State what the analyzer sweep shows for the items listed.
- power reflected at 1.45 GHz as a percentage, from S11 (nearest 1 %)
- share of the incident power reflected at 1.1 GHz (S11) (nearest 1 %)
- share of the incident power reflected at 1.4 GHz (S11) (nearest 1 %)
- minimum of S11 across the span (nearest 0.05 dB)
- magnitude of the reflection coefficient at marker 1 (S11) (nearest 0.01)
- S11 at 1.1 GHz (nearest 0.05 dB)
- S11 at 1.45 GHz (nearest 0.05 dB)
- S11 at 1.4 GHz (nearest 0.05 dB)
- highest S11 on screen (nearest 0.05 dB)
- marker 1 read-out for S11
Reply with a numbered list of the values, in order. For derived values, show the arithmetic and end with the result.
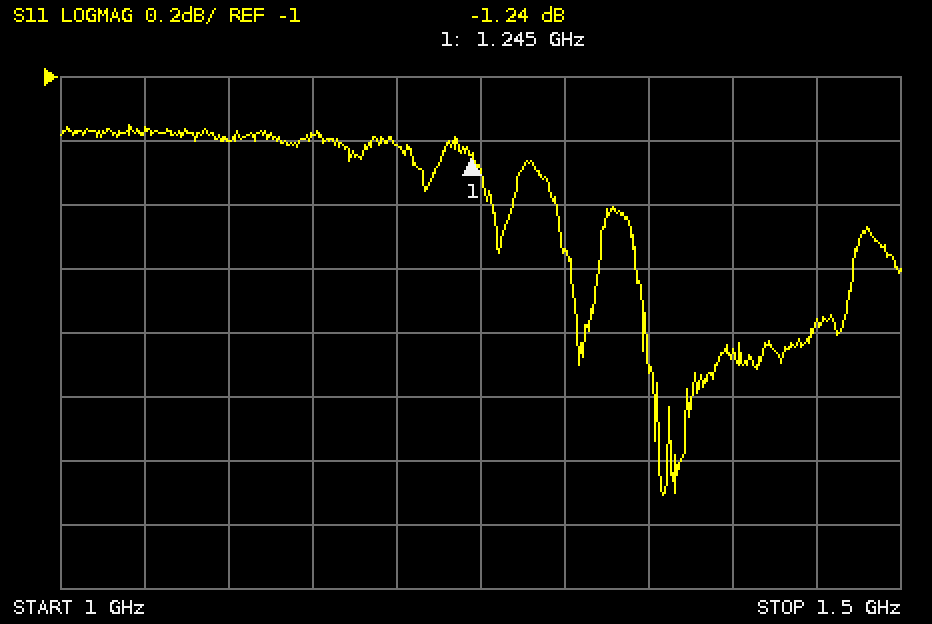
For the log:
1. 10^(-1.75/10) ≈ 67 %
2. 10^(-1.2/10) ≈ 76 %
3. 10^(-1.85/10) ≈ 65 %
4. -2.30 dB
5. 10^(-1.24/20) ≈ 0.87
6. -1.20 dB
7. -1.75 dB
8. -1.85 dB
9. -1.15 dB
10. -1.24 dB
